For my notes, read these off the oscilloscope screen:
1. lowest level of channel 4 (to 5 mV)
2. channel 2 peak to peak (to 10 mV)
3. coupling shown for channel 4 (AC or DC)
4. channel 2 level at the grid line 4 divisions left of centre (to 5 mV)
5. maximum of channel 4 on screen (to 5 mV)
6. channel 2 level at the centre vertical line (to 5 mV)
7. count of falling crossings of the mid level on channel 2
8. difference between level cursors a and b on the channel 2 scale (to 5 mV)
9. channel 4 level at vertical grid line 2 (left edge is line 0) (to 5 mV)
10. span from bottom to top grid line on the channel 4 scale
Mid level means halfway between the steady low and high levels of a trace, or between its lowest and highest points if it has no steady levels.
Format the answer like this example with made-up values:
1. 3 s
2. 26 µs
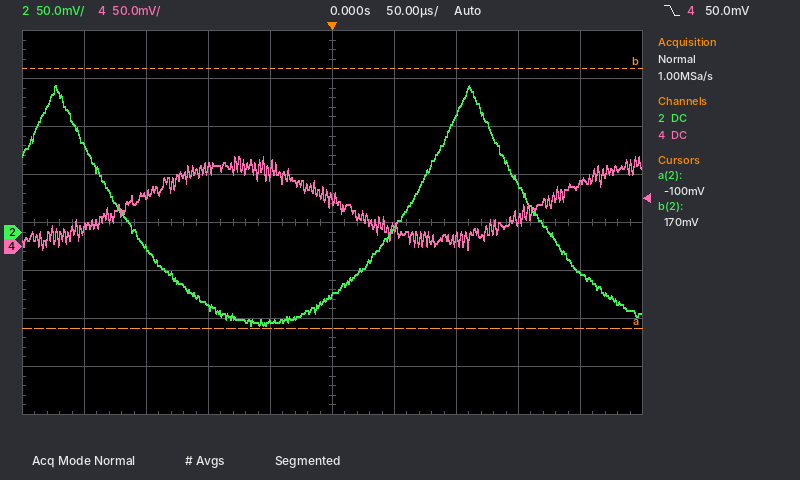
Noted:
1. -5 mV
2. 250 mV
3. DC
4. 90 mV
5. 95 mV
6. -65 mV
7. 2
8. 270 mV
9. 55 mV
10. 400 mV
